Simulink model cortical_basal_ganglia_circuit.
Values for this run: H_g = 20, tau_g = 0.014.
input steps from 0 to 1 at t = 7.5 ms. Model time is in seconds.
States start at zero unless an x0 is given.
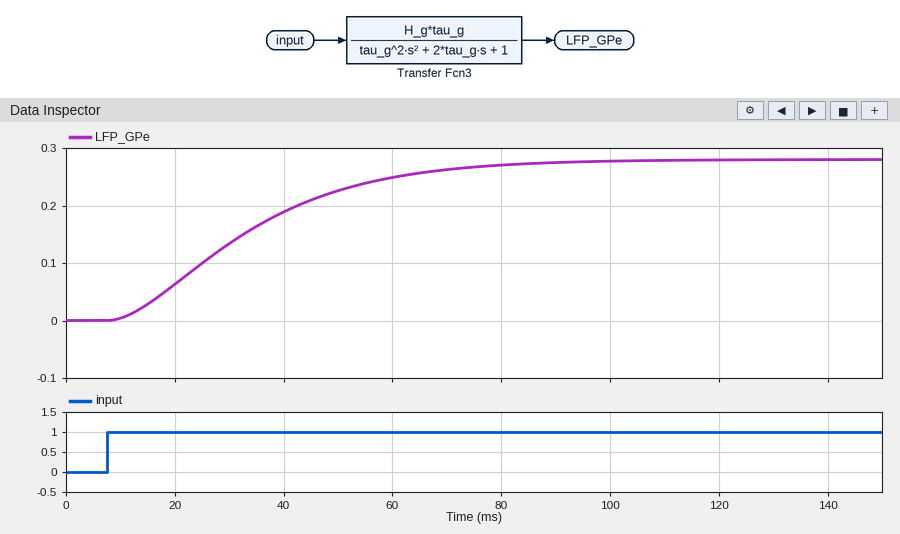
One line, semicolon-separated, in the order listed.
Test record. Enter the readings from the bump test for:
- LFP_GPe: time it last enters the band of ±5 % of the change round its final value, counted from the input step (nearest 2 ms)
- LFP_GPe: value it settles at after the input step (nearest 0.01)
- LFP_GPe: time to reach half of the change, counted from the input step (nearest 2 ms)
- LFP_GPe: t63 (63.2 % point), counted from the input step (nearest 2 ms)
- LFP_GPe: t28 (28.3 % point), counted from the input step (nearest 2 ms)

66 ms; 0.28; 24 ms; 30 ms; 14 ms
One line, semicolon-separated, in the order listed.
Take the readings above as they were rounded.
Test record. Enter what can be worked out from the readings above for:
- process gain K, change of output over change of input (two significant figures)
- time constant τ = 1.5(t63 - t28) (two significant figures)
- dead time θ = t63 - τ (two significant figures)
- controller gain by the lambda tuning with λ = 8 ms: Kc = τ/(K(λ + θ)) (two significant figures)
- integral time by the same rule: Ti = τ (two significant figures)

0.28; 24 ms; 6.0 ms; 6.1; 24 ms
